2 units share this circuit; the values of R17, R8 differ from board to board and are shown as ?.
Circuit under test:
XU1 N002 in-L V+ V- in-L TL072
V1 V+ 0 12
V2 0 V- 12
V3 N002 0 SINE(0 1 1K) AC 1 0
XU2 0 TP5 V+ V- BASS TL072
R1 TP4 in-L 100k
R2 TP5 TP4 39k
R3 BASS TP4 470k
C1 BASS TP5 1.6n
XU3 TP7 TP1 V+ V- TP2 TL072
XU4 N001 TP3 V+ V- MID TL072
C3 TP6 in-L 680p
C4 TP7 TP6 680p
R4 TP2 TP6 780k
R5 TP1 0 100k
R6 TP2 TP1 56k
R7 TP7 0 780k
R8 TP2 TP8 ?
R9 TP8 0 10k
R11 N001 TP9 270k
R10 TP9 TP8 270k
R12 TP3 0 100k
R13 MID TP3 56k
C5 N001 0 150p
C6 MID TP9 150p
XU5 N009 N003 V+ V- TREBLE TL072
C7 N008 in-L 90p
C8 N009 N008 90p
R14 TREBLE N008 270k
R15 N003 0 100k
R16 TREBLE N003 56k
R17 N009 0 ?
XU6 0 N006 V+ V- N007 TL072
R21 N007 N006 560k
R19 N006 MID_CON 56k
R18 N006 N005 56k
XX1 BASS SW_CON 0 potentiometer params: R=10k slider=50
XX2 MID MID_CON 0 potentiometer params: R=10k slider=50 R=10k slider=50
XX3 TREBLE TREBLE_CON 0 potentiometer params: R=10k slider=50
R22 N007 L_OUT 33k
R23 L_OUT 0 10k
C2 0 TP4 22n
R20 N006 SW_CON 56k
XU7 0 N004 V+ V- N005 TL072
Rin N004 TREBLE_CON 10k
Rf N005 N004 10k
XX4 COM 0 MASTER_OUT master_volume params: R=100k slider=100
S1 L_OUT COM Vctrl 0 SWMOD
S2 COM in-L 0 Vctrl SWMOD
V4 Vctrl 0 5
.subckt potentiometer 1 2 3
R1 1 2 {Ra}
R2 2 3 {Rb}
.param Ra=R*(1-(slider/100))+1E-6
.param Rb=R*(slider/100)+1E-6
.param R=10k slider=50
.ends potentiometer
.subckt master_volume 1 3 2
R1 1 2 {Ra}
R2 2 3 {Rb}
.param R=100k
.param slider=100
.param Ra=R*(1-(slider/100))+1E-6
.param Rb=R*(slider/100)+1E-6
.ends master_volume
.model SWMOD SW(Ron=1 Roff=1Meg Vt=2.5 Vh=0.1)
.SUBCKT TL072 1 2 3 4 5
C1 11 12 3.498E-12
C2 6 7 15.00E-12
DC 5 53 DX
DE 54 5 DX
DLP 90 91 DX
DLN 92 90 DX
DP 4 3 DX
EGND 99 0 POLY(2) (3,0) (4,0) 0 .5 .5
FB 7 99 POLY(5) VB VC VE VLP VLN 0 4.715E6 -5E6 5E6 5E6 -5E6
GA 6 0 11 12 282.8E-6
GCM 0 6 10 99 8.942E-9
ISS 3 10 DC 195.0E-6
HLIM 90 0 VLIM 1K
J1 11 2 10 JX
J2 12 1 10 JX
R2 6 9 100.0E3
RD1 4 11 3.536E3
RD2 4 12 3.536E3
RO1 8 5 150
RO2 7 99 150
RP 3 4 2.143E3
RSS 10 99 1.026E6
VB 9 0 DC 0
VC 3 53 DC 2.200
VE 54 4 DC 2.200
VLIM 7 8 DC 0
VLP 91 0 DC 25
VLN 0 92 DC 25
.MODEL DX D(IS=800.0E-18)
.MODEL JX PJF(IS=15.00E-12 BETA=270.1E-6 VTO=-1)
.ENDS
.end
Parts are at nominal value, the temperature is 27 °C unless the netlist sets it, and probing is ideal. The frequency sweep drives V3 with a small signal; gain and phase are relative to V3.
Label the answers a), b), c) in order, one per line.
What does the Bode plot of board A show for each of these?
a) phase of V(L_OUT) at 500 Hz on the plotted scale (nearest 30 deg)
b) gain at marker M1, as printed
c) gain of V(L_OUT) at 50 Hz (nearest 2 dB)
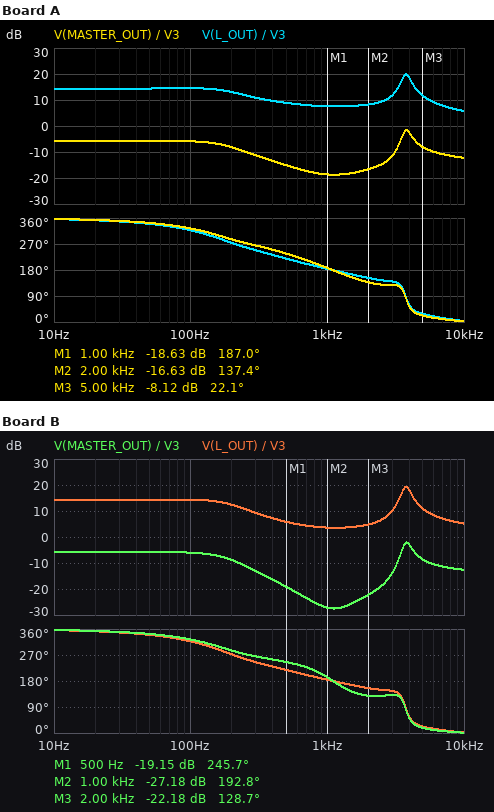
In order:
a) 210 deg
b) -18.63 dB
c) 14 dB
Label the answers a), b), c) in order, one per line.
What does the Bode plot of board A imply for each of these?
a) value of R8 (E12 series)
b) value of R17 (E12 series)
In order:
a) 2.7 kΩ
b) 820 kΩ
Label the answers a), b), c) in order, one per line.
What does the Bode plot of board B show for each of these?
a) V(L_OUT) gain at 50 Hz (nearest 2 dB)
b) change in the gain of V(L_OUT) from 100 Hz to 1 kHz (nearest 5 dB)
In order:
a) 14 dB
b) -10 dB
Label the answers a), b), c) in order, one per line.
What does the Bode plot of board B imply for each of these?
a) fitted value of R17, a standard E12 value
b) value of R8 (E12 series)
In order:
a) 820 kΩ
b) 12 kΩ
